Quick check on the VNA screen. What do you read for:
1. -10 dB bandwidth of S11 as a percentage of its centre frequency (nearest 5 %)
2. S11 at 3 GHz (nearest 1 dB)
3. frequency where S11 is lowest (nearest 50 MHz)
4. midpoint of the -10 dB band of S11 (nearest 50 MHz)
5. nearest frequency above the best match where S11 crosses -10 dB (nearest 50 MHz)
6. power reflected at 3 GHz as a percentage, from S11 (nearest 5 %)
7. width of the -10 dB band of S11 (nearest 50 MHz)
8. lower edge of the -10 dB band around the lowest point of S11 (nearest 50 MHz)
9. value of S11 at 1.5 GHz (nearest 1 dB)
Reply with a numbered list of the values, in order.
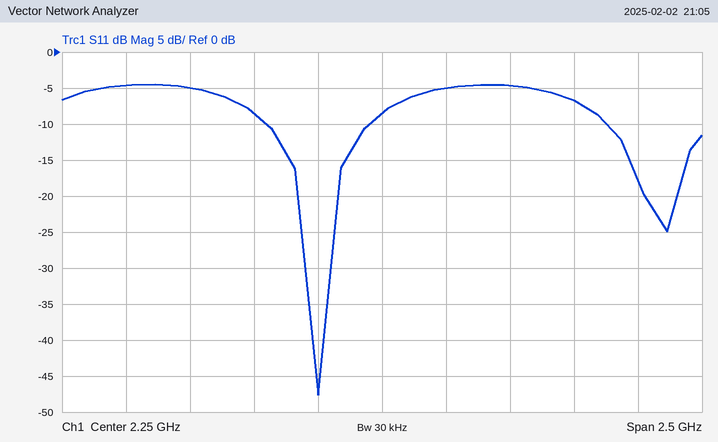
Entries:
1. 20 %
2. -7 dB
3. 2.00 GHz
4. 2.00 GHz
5. 2.20 GHz
6. 20 %
7. 400 MHz
8. 1.80 GHz
9. -5 dB
